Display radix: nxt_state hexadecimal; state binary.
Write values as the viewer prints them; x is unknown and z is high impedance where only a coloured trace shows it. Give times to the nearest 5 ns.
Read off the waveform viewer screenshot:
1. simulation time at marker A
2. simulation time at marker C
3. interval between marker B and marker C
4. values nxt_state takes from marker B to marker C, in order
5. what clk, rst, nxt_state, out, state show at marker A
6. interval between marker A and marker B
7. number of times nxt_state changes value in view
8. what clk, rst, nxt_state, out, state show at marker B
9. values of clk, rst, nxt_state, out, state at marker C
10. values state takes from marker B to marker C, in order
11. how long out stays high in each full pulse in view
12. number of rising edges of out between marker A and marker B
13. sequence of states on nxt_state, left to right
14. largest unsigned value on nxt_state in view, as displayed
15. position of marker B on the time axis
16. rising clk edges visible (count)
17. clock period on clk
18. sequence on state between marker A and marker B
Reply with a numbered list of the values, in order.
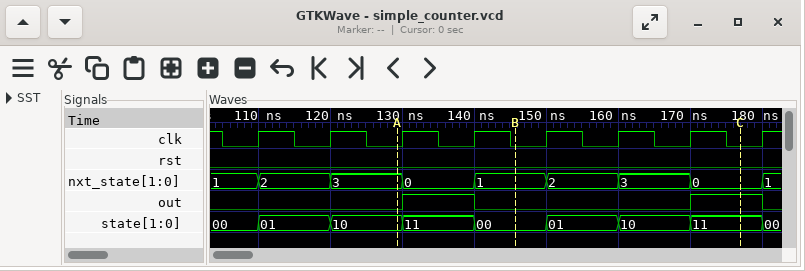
1. 130 ns
2. 175 ns
3. 30 ns
4. 1, 2, 3, 0
5. clk=0, rst=0, nxt_state=3, out=0, state=10
6. 15 ns
7. 8
8. clk=0, rst=0, nxt_state=1, out=0, state=00
9. clk=0, rst=0, nxt_state=0, out=1, state=11
10. 00, 01, 10, 11
11. 10 ns, 10 ns
12. 1
13. 1, 2, 3, 0, 1, 2, 3, 0, 1
14. 3
15. 145 ns
16. 8
17. 10 ns
18. 10, 11, 00
